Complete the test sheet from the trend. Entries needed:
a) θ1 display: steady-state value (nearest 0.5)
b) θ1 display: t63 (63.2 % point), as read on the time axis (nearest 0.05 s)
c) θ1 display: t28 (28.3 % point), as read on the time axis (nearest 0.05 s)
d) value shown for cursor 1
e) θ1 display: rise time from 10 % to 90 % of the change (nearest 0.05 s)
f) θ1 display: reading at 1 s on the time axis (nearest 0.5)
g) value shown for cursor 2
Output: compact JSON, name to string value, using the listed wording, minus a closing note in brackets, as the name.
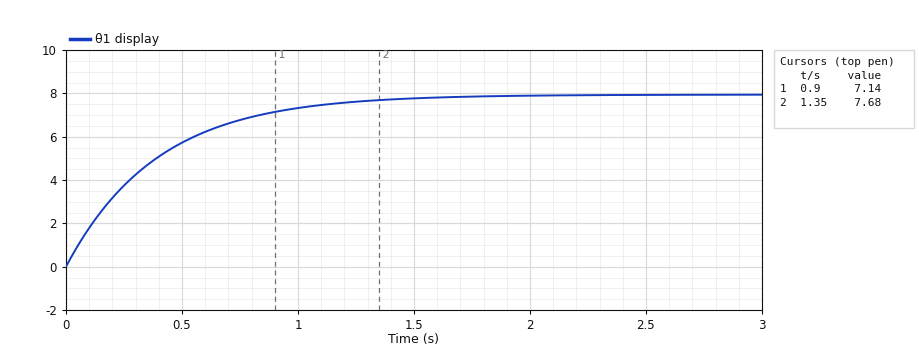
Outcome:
{"θ1 display: steady-state value": "8.0", "θ1 display: t63 (63.2 % point), as read on the time axis": "0.40 s", "θ1 display: t28 (28.3 % point), as read on the time axis": "0.15 s", "value shown for cursor 1": "7.14", "θ1 display: rise time from 10 % to 90 % of the change": "0.85 s", "θ1 display: reading at 1 s on the time axis": "7.5", "value shown for cursor 2": "7.68"}
